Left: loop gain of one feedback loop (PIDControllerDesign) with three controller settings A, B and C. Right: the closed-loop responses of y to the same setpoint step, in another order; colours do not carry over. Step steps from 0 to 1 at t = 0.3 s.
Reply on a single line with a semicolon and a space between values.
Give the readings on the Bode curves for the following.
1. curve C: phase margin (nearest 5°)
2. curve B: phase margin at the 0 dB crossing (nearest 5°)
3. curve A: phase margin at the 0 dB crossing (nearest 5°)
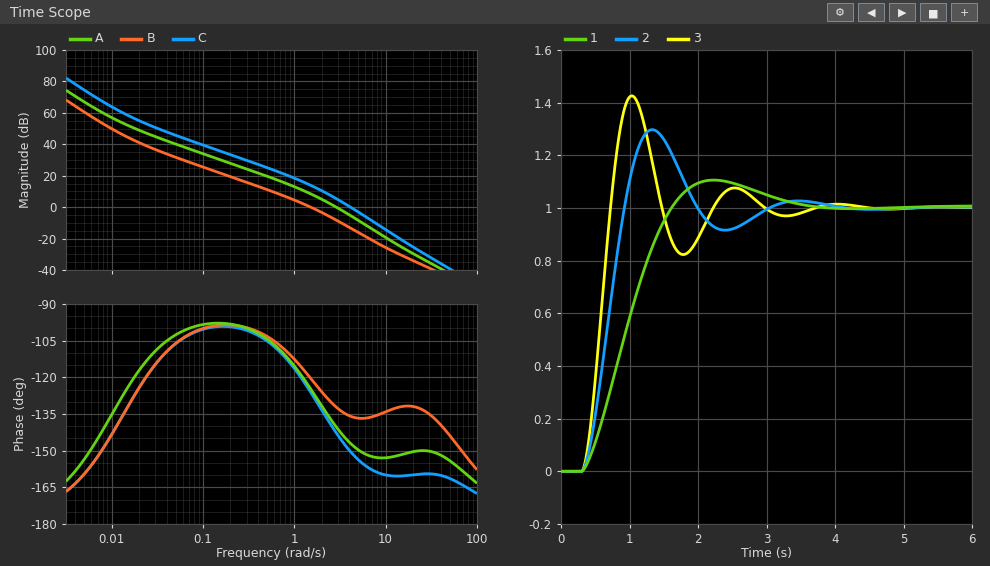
30°; 60°; 40°
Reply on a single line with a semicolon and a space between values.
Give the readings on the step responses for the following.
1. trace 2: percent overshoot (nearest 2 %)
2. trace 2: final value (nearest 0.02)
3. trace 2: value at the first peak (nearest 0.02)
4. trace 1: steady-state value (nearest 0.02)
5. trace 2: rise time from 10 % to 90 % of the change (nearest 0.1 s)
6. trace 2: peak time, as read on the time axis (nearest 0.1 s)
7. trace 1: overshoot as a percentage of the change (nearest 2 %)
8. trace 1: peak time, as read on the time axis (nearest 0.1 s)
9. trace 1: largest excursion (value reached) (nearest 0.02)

30 %; 1.00; 1.30; 1.00; 0.4 s; 1.3 s; 10 %; 2.2 s; 1.10
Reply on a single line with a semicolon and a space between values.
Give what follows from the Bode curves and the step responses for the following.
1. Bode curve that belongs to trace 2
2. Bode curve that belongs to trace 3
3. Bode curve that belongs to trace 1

A; C; B
